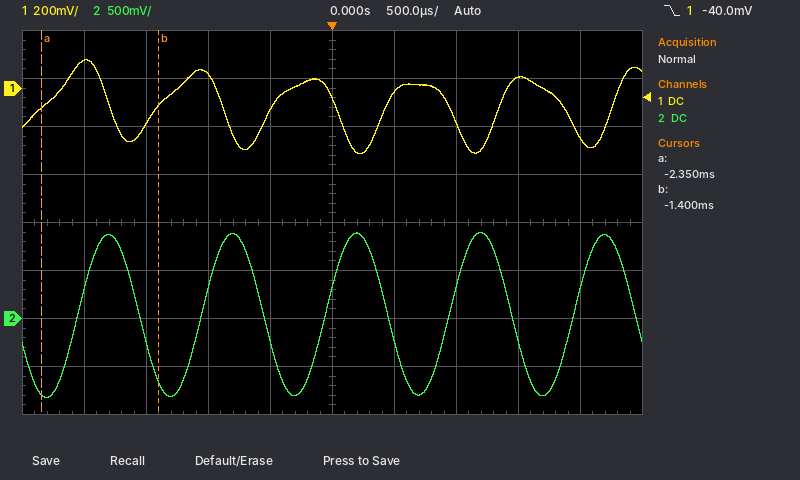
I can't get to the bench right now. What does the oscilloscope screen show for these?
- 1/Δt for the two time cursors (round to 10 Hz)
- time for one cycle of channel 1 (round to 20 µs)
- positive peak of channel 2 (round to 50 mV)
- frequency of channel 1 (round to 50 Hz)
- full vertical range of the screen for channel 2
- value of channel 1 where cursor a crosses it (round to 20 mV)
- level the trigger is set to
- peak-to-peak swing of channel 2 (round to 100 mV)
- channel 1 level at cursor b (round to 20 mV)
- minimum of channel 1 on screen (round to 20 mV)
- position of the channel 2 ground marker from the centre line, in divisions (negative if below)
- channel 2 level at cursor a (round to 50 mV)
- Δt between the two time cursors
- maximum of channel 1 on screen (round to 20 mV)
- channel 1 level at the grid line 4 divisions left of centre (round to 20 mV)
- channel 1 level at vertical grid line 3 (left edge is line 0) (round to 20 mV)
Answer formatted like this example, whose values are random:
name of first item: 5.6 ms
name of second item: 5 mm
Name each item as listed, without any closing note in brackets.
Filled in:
1/Δt for the two time cursors: 1.05 kHz
time for one cycle of channel 1: 920 µs
positive peak of channel 2: 900 mV
frequency of channel 1: 1.10 kHz
full vertical range of the screen for channel 2: 4 V
value of channel 1 where cursor a crosses it: -80 mV
level the trigger is set to: -40.0 mV
peak-to-peak swing of channel 2: 1.70 V
channel 1 level at cursor b: -80 mV
minimum of channel 1 on screen: -280 mV
position of the channel 2 ground marker from the centre line, in divisions: -2.0 div
channel 2 level at cursor a: -800 mV
Δt between the two time cursors: 950 µs
maximum of channel 1 on screen: 120 mV
channel 1 level at the grid line 4 divisions left of centre: 120 mV
channel 1 level at vertical grid line 3 (left edge is line 0): 60 mV
